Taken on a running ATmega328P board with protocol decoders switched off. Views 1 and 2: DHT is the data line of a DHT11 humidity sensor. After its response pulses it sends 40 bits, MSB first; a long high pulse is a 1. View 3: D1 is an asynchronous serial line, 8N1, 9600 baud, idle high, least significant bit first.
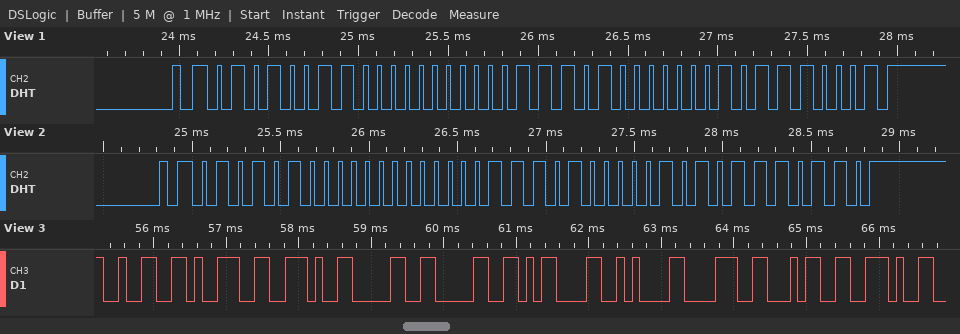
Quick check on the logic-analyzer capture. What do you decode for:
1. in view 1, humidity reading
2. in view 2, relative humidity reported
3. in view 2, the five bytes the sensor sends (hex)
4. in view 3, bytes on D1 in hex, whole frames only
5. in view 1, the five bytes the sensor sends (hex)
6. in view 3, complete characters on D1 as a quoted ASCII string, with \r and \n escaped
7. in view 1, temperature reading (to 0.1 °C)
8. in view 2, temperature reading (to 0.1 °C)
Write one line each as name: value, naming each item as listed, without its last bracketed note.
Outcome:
in view 1, humidity reading: 83 %
in view 2, relative humidity reported: 84 %
in view 2, the five bytes the sensor sends: 54 00 1D 05 76
in view 3, bytes on D1 in hex, whole frames only: 32 39 2E 30 30 0D 0A 38 34 2E
in view 1, the five bytes the sensor sends: 53 00 1D 01 71
in view 3, complete characters on D1 as a quoted ASCII string, with \r and \n escaped: "29.00\r\n84."
in view 1, temperature reading: 29.1 °C
in view 2, temperature reading: 29.5 °C
